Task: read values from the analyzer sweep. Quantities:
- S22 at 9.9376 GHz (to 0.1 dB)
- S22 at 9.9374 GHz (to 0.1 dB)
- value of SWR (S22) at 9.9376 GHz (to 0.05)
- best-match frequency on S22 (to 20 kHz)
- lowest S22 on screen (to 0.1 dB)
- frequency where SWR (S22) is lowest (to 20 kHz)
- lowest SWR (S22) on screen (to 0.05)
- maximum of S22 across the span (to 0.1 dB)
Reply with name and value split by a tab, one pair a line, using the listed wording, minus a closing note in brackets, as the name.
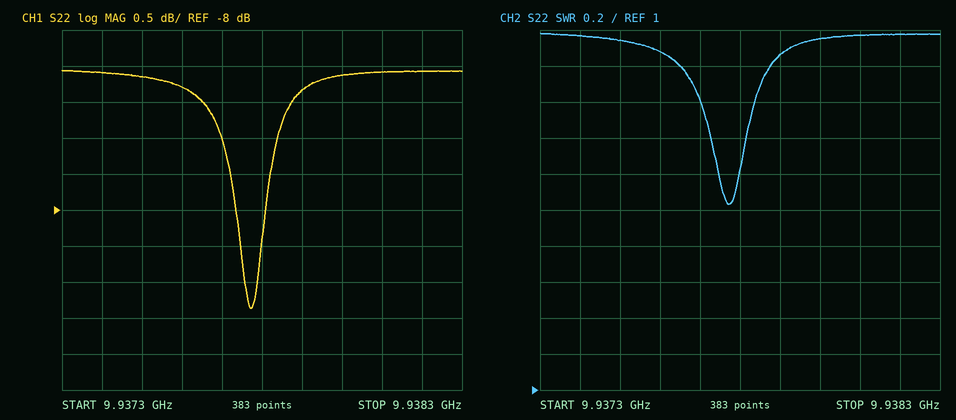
S22 at 9.9376 GHz	-6.3 dB
S22 at 9.9374 GHz	-6.1 dB
value of SWR (S22) at 9.9376 GHz	2.90
best-match frequency on S22	9.93778 GHz
lowest S22 on screen	-9.4 dB
frequency where SWR (S22) is lowest	9.93778 GHz
lowest SWR (S22) on screen	2.05
maximum of S22 across the span	-6.1 dB
